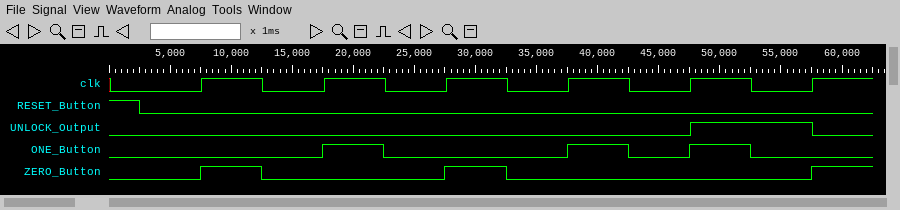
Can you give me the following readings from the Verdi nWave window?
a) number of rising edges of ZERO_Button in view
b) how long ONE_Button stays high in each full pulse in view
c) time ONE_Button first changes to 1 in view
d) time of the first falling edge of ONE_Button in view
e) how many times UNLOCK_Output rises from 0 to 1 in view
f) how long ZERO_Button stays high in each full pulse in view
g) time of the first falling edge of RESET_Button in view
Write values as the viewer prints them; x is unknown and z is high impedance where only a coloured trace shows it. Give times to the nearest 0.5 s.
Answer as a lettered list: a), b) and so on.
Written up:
a) 3
b) 5 s, 5 s, 5 s
c) 17.5 s
d) 22.5 s
e) 1
f) 5 s, 5 s
g) 2.5 s
